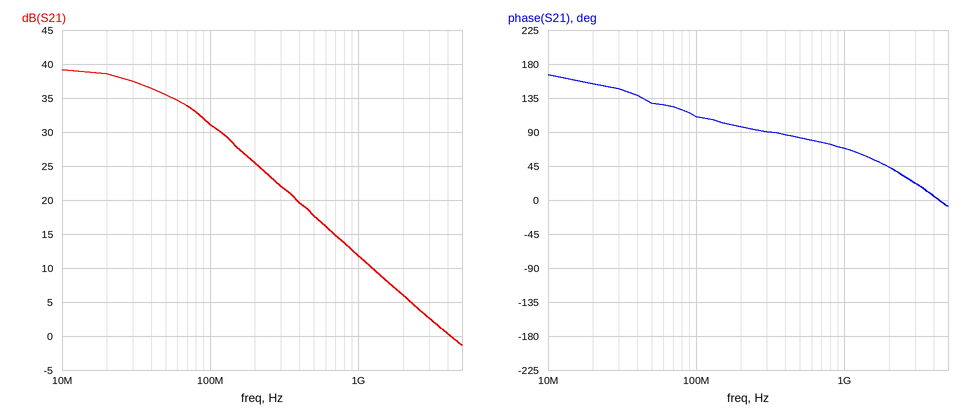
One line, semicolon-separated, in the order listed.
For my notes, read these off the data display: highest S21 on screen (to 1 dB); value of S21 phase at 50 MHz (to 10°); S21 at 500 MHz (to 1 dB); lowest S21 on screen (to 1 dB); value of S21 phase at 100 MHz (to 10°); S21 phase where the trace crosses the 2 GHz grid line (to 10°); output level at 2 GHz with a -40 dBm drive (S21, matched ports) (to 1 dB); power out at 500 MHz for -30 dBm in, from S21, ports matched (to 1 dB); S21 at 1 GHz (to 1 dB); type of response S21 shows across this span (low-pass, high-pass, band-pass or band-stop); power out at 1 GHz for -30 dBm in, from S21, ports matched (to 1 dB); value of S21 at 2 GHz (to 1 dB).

39 dB; 130°; 18 dB; -1 dB; 110°; 40°; -34 dBm; -12 dBm; 12 dB; low-pass; -18 dBm; 6 dB
